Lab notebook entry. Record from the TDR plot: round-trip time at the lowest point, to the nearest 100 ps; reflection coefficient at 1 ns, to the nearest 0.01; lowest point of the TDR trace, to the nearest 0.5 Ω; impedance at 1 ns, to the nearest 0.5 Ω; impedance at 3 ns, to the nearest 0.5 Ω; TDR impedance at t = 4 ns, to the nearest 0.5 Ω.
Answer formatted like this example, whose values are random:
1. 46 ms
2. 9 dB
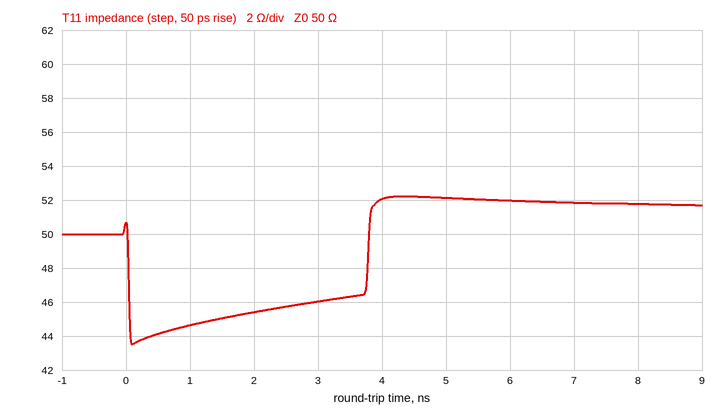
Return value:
1. 100 ps
2. -0.06
3. 43.5 Ω
4. 44.5 Ω
5. 46.0 Ω
6. 52.0 Ω
